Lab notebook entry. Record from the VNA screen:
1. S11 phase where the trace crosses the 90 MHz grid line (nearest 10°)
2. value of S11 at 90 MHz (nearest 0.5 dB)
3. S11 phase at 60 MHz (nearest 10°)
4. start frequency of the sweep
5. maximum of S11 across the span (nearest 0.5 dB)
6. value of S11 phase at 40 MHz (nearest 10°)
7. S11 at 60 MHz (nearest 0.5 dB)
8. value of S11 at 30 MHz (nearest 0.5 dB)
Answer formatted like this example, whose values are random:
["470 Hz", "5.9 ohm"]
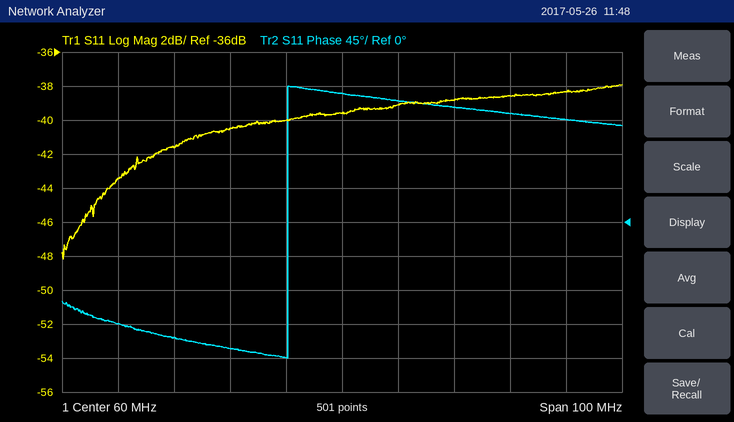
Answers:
["140°", "-38.5 dB", "170°", "10 MHz", "-38.0 dB", "-170°", "-39.5 dB", "-41.5 dB"]
